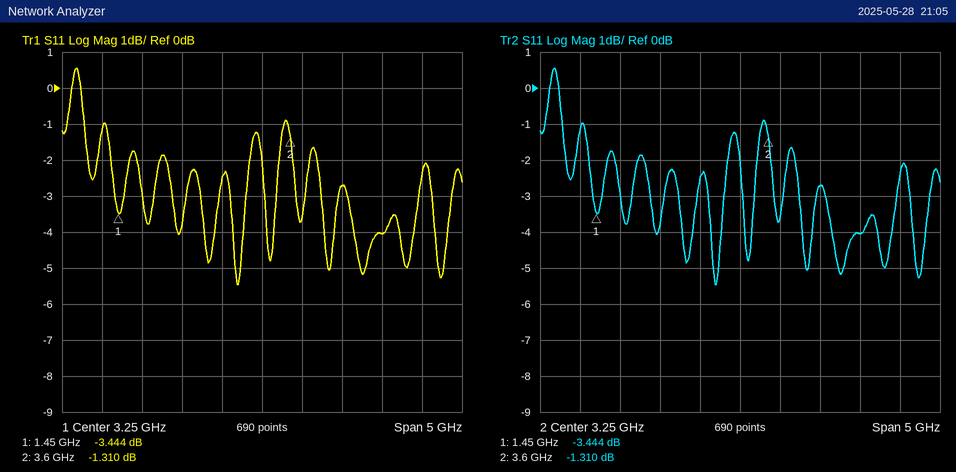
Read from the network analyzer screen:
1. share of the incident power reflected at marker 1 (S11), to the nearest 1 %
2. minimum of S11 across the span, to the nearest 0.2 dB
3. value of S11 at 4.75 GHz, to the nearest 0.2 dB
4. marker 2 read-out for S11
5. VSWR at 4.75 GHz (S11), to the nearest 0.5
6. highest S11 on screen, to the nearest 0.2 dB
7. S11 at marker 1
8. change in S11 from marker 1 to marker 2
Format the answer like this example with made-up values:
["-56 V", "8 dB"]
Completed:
["45 %", "-5.4 dB", "-4.0 dB", "-1.310 dB", "4.5", "0.6 dB", "-3.444 dB", "2.134 dB"]
